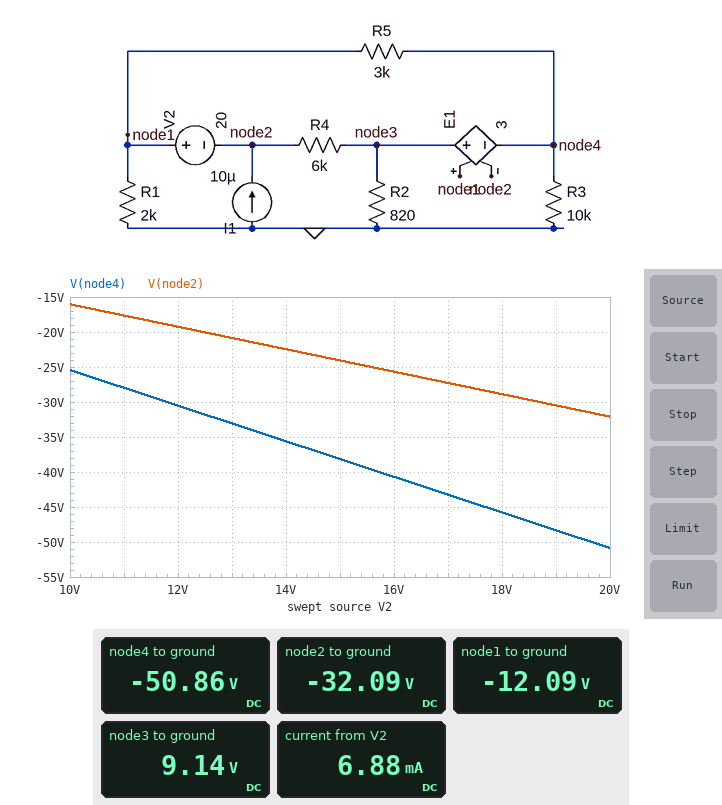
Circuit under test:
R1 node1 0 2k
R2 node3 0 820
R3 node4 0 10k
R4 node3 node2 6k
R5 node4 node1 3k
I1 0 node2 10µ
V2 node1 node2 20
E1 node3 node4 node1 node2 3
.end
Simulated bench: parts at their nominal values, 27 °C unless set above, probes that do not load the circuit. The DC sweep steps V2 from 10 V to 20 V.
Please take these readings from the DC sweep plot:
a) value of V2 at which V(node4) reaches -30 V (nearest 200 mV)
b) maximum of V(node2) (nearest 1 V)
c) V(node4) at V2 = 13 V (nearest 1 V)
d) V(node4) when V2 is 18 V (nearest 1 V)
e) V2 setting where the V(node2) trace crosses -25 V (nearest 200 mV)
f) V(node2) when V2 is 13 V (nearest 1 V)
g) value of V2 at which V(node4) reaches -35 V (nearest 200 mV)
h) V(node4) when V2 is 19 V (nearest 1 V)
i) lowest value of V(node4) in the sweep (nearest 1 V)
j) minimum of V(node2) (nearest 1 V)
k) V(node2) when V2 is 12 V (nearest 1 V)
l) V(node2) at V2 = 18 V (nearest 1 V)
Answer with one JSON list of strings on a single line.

["11.8 V", "-16 V", "-33 V", "-46 V", "15.6 V", "-21 V", "13.8 V", "-48 V", "-51 V", "-32 V", "-19 V", "-29 V"]
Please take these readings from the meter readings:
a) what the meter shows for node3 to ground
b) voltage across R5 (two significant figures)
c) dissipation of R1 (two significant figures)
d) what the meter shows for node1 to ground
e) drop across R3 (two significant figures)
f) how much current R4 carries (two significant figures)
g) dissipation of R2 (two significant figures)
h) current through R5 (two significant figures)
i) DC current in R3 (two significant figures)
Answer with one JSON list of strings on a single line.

["9.14 V", "39 V", "73 mW", "-12.09 V", "51 V", "6.9 mA", "100 mW", "13 mA", "5.1 mA"]
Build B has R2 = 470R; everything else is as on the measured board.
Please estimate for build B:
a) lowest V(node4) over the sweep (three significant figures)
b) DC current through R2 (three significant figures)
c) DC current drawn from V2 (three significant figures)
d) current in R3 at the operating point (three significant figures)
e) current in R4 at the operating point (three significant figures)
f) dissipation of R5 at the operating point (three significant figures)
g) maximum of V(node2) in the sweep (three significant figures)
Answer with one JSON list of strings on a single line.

["-54.2 V", "12.3 mA", "6.60 mA", "5.42 mA", "6.59 mA", "545 mW", "-16.9 V"]
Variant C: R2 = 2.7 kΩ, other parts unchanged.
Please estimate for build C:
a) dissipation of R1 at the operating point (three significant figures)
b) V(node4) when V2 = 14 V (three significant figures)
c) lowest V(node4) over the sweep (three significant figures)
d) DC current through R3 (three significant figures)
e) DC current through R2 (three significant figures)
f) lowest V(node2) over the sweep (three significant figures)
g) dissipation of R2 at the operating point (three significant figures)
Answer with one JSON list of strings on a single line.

["22.5 mW", "-28.1 V", "-40.1 V", "4.01 mA", "7.37 mA", "-26.7 V", "147 mW"]
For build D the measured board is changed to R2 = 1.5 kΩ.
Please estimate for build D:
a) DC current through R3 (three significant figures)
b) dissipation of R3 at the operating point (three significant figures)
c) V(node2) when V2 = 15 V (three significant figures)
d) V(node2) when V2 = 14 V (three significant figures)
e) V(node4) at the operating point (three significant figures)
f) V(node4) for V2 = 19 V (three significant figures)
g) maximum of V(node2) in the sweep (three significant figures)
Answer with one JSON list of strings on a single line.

["4.59 mA", "211 mW", "-22.2 V", "-20.7 V", "-45.9 V", "-43.6 V", "-14.8 V"]
